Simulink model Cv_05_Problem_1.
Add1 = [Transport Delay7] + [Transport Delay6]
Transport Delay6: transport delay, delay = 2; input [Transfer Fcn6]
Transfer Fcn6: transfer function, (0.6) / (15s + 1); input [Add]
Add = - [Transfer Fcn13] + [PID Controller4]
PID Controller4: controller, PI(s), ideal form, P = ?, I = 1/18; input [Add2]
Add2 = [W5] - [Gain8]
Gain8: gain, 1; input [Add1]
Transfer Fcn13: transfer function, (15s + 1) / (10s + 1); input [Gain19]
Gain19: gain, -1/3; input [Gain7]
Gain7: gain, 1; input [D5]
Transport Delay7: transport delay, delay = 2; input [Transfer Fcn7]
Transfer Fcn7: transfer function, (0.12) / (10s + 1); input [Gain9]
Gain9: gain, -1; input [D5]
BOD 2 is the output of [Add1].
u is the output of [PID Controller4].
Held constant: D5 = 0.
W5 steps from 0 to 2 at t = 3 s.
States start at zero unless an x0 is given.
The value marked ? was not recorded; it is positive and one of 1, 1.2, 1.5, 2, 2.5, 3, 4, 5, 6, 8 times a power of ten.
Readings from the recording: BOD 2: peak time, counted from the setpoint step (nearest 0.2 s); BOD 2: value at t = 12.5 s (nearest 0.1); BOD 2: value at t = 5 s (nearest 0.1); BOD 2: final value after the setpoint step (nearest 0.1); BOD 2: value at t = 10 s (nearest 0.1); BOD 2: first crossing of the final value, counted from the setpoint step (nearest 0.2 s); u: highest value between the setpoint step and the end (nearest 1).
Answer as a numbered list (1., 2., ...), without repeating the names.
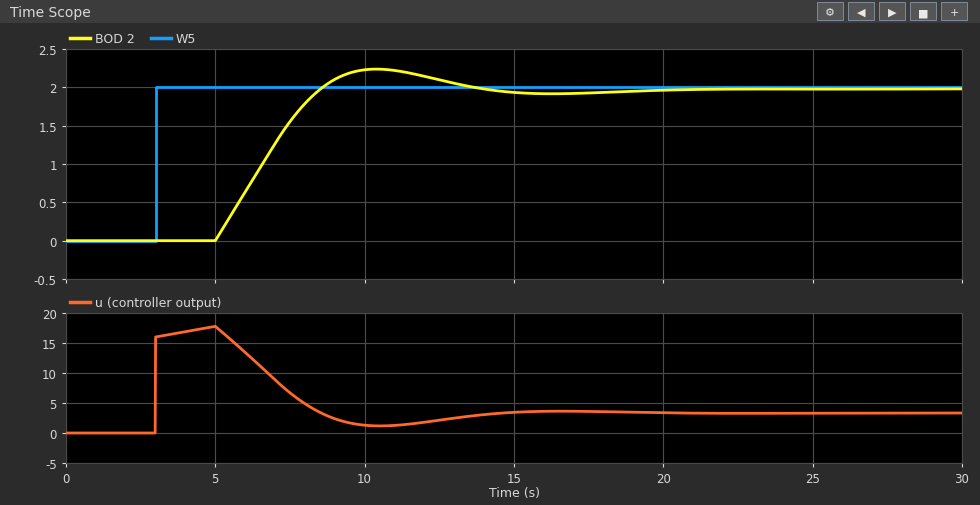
1. 7.4 s
2. 2.1
3. 0.0
4. 2.0
5. 2.2
6. 5.6 s
7. 18
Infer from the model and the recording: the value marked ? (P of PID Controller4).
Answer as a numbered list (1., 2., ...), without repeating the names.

1. 8
